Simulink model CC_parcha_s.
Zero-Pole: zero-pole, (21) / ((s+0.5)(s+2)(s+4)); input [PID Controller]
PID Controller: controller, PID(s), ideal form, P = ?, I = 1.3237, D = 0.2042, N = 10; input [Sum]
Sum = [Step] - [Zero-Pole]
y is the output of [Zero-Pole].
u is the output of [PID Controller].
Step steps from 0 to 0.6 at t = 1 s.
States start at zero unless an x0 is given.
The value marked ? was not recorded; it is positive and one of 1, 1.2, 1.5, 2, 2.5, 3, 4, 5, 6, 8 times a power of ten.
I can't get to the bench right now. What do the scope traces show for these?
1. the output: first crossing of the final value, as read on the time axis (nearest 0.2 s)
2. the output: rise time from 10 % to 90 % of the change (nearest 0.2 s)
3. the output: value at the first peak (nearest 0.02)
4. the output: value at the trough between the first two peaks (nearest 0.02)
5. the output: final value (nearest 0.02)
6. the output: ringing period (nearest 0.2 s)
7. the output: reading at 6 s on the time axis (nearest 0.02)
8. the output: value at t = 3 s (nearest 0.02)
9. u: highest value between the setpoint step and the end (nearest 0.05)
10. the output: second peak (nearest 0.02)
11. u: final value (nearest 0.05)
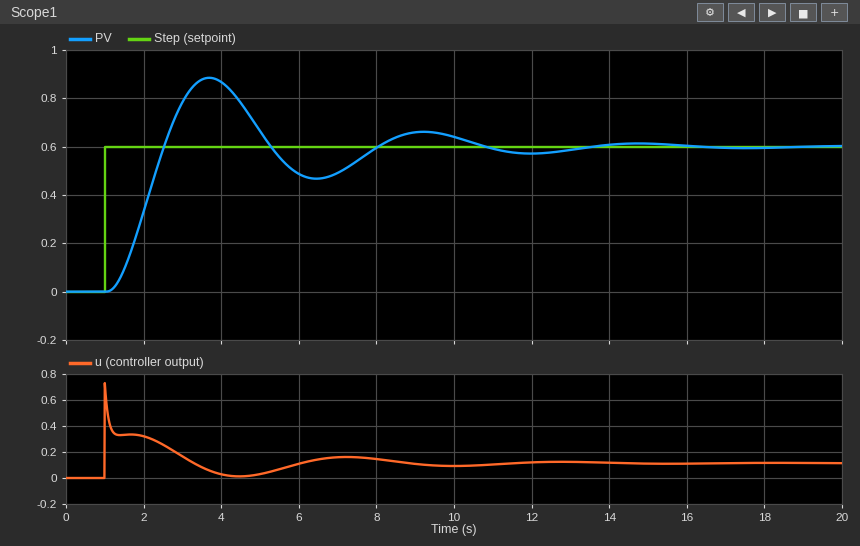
2.6 s
1.0 s
0.88
0.46
0.60
5.6 s
0.48
0.78
0.75
0.66
0.10
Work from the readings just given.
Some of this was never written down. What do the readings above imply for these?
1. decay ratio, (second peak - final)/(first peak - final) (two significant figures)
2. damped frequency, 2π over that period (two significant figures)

0.21
1.1 rad/s
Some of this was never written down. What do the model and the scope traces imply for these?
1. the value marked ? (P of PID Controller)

0.4
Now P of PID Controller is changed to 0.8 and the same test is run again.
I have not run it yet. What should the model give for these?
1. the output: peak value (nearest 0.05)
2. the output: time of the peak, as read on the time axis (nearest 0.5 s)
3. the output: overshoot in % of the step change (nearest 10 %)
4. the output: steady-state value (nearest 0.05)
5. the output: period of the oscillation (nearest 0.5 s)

0.95
3.0 s
60 %
0.60
4.0 s
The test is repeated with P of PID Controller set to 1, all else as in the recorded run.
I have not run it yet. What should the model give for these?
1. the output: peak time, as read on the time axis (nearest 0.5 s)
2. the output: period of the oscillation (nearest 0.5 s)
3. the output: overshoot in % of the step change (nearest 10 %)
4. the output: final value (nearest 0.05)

2.5 s
3.5 s
60 %
0.60
